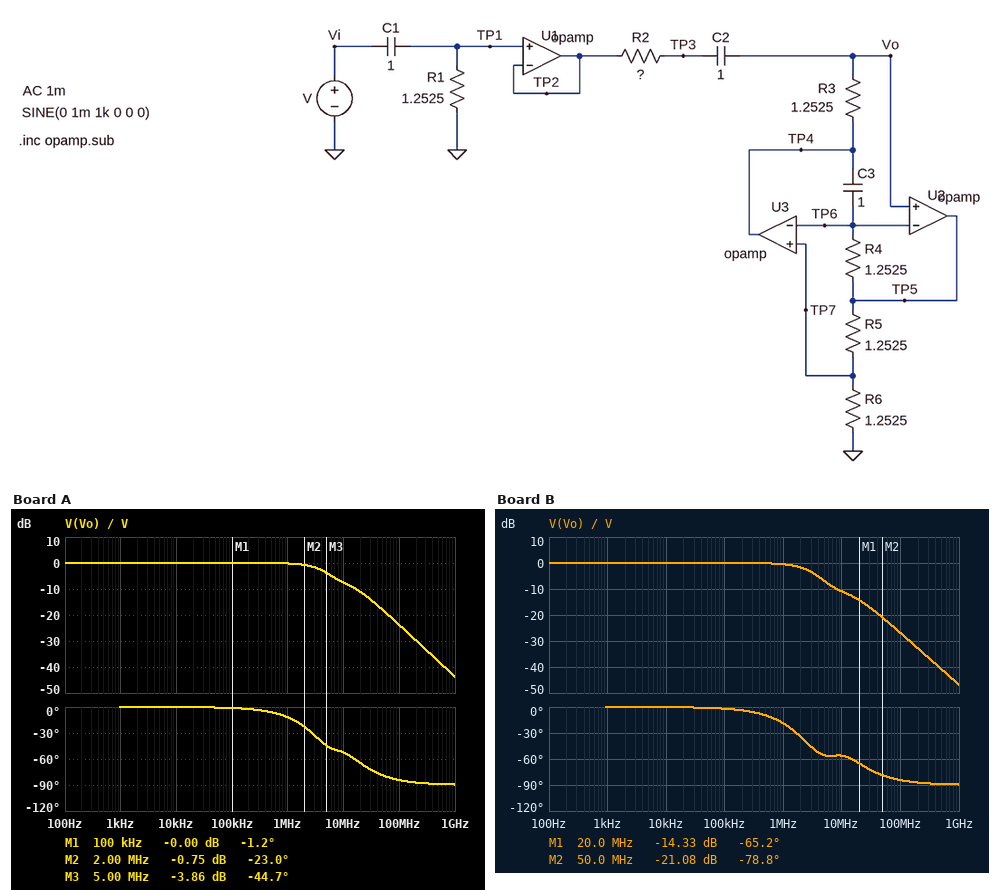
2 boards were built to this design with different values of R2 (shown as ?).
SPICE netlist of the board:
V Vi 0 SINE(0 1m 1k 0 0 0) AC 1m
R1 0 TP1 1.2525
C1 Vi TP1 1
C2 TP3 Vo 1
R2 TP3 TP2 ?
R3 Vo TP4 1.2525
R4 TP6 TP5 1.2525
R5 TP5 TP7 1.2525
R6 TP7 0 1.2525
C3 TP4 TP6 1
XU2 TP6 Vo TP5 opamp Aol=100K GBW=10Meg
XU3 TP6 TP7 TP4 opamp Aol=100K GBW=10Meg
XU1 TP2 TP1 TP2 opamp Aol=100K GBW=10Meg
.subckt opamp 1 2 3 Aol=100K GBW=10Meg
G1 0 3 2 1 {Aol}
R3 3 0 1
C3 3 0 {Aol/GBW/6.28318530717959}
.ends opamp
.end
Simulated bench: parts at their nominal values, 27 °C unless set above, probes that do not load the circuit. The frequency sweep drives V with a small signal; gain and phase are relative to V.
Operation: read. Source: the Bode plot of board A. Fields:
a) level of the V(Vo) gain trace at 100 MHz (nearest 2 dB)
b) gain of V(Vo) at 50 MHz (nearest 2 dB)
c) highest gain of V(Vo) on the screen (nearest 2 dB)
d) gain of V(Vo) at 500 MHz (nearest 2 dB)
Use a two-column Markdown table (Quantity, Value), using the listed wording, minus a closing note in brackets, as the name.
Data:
| Quantity | Value |
|---|---|
| level of the V(Vo) gain trace at 100 MHz | -24 dB |
| gain of V(Vo) at 50 MHz | -18 dB |
| highest gain of V(Vo) on the screen | 0 dB |
| gain of V(Vo) at 500 MHz | -38 dB |
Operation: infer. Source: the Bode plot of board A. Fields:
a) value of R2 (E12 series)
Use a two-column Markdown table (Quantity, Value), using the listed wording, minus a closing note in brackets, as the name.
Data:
| Quantity | Value |
|---|---|
| value of R2 | 0.68 Ω |
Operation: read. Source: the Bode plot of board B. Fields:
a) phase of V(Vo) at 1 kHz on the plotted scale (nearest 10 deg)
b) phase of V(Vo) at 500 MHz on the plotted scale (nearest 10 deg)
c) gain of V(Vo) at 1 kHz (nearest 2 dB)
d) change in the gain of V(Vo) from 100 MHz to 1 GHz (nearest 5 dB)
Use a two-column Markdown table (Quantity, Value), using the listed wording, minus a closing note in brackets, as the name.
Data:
| Quantity | Value |
|---|---|
| phase of V(Vo) at 1 kHz on the plotted scale | 0 deg |
| phase of V(Vo) at 500 MHz on the plotted scale | -90 deg |
| gain of V(Vo) at 1 kHz | 0 dB |
| change in the gain of V(Vo) from 100 MHz to 1 GHz | -20 dB |
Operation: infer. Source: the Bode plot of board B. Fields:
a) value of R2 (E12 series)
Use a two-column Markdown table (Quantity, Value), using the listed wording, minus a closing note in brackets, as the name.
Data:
| Quantity | Value |
|---|---|
| value of R2 | 1.5 Ω |
